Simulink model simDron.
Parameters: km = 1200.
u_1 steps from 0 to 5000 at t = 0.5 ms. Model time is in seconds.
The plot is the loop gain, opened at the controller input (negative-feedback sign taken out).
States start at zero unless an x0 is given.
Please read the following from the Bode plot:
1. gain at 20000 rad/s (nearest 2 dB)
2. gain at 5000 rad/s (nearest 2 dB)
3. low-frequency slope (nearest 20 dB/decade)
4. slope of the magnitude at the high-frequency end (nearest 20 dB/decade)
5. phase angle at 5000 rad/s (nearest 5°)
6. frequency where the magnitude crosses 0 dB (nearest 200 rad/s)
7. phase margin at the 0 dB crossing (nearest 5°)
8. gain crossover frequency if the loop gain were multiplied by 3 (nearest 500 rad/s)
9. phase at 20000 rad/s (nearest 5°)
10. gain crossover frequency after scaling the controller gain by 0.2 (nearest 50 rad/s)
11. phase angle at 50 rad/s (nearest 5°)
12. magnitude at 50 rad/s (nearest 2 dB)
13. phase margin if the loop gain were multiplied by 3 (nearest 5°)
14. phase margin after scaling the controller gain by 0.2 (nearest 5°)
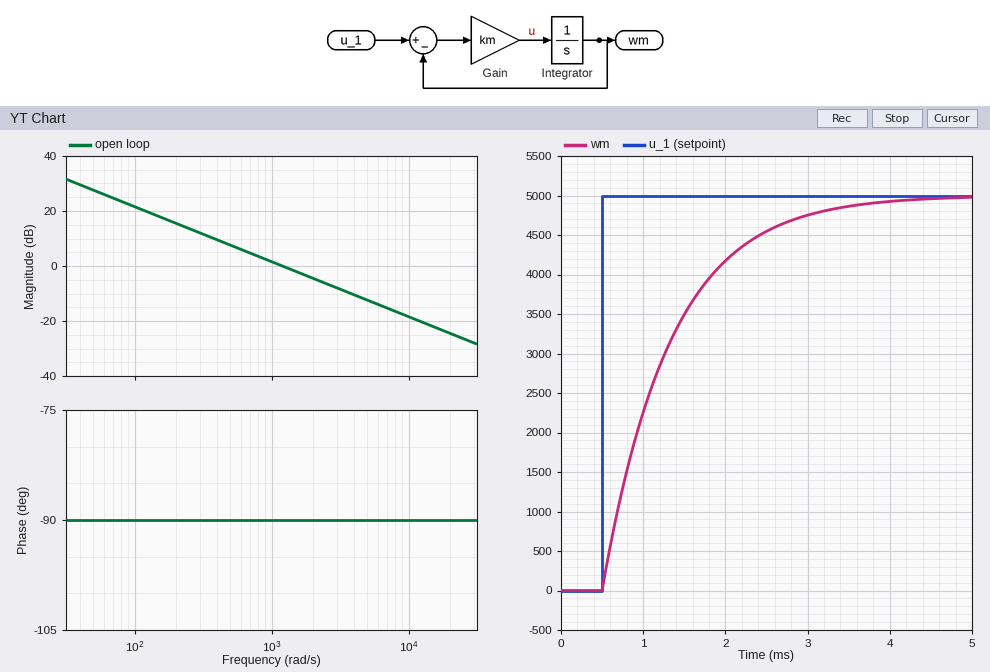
-24 dB
-12 dB
-20 dB/decade
-20 dB/decade
-90°
1200 rad/s
90°
3500 rad/s
-90°
250 rad/s
-90°
28 dB
90°
90°
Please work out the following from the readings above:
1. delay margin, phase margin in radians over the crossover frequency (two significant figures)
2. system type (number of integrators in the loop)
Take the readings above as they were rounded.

0.0013 s
1
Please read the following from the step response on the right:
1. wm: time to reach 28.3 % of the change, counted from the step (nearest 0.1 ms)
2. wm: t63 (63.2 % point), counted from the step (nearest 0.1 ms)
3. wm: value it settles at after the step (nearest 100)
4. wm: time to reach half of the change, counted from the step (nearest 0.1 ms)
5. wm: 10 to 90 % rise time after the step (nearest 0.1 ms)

0.3 ms
0.8 ms
5000
0.6 ms
1.8 ms
